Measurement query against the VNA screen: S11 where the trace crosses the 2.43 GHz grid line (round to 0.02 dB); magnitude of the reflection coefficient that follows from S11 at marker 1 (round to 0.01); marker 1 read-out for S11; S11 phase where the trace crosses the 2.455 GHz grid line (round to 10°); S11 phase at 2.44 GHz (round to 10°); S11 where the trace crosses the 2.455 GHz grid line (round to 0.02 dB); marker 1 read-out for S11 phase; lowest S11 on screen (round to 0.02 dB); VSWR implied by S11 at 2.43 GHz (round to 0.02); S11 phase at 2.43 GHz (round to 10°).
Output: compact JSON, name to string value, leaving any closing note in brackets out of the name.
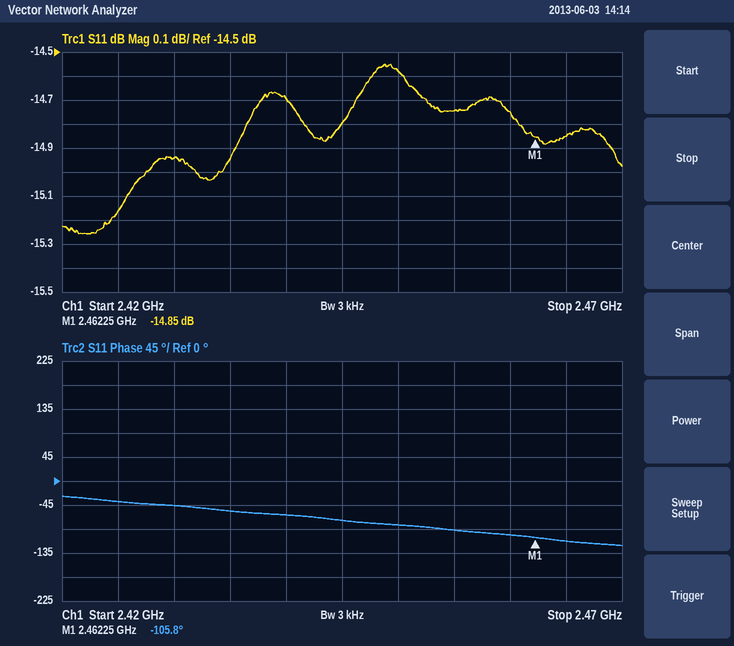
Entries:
{"S11 where the trace crosses the 2.43 GHz grid line": "-14.94 dB", "magnitude of the reflection coefficient that follows from S11 at marker 1": "0.18", "marker 1 read-out for S11": "-14.85 dB", "S11 phase where the trace crosses the 2.455 GHz grid line": "-90°", "S11 phase at 2.44 GHz": "-60°", "S11 where the trace crosses the 2.455 GHz grid line": "-14.74 dB", "marker 1 read-out for S11 phase": "-105.8°", "lowest S11 on screen": "-15.26 dB", "VSWR implied by S11 at 2.43 GHz": "1.44", "S11 phase at 2.43 GHz": "-50°"}
